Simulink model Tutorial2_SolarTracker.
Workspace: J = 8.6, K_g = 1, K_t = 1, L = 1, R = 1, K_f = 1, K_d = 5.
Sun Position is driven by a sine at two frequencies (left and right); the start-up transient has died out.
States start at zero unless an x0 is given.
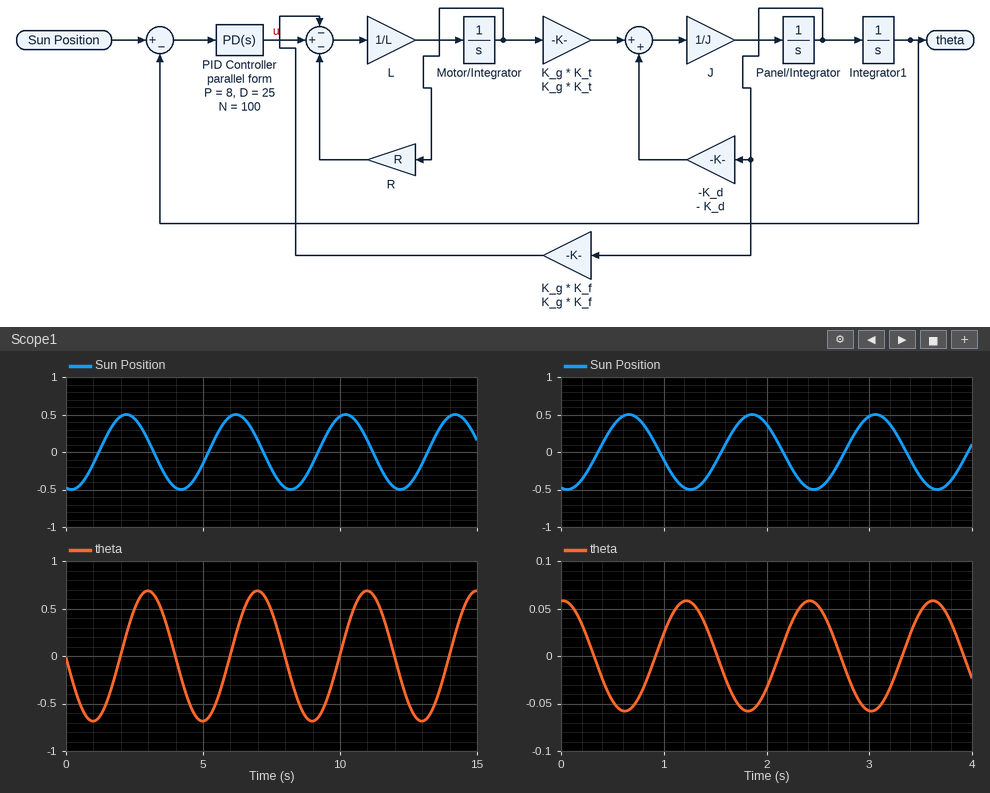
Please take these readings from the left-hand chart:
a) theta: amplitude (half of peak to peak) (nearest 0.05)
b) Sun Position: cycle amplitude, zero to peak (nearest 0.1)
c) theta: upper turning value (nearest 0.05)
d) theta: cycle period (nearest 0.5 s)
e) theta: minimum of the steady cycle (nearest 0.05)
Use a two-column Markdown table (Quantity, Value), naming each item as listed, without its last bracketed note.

| Quantity | Value |
|---|---|
| theta: amplitude (half of peak to peak) | 0.70 |
| Sun Position: cycle amplitude, zero to peak | 0.5 |
| theta: upper turning value | 0.70 |
| theta: cycle period | 4.0 s |
| theta: minimum of the steady cycle | -0.70 |
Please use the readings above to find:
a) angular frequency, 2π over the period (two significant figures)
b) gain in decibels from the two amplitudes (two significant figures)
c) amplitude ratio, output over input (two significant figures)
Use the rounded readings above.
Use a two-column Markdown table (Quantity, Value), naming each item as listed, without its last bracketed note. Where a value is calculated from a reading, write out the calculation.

| Quantity | Value |
|---|---|
| angular frequency, 2π over the period | 2π / 4 = 1.6 rad/s |
| gain in decibels from the two amplitudes | 20 log10(0.7 / 0.5) = 2.9 dB |
| amplitude ratio, output over input | 0.7 / 0.5 = 1.4 |
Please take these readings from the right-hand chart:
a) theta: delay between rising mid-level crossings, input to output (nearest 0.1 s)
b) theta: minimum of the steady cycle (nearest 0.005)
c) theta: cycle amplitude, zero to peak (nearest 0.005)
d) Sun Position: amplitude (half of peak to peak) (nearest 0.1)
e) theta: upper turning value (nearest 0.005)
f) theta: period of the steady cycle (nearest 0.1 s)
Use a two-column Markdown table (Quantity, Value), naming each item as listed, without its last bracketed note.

| Quantity | Value |
|---|---|
| theta: delay between rising mid-level crossings, input to output | 0.6 s |
| theta: minimum of the steady cycle | -0.060 |
| theta: cycle amplitude, zero to peak | 0.060 |
| Sun Position: amplitude (half of peak to peak) | 0.5 |
| theta: upper turning value | 0.060 |
| theta: period of the steady cycle | 1.2 s |
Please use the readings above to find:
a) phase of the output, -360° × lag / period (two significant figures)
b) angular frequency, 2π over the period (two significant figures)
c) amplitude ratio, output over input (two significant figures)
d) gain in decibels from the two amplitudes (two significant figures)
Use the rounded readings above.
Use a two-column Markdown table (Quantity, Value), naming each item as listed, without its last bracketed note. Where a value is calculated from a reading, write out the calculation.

| Quantity | Value |
|---|---|
| phase of the output, -360° × lag / period | -360 × 0.6 / 1.2 = -180° |
| angular frequency, 2π over the period | 2π / 1.2 = 5.2 rad/s |
| amplitude ratio, output over input | 0.06 / 0.5 = 0.12 |
| gain in decibels from the two amplitudes | 20 log10(0.06 / 0.5) = -18 dB |
